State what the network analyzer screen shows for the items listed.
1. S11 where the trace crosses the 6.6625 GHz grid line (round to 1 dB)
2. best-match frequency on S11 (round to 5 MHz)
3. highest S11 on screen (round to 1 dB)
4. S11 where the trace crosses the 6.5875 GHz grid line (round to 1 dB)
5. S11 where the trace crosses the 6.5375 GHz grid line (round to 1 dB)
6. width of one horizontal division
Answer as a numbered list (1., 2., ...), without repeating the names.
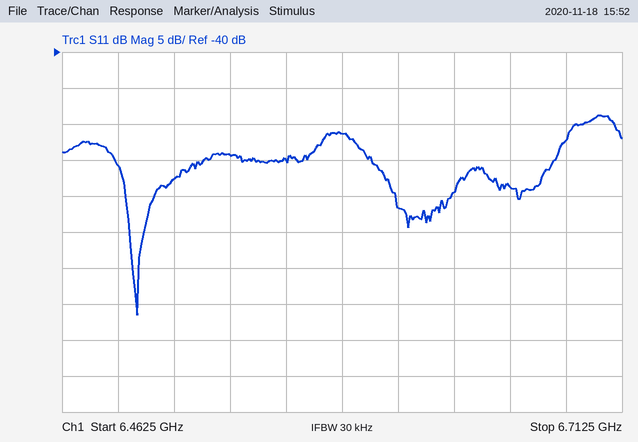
1. -59 dB
2. 6.495 GHz
3. -49 dB
4. -51 dB
5. -54 dB
6. 25 MHz
